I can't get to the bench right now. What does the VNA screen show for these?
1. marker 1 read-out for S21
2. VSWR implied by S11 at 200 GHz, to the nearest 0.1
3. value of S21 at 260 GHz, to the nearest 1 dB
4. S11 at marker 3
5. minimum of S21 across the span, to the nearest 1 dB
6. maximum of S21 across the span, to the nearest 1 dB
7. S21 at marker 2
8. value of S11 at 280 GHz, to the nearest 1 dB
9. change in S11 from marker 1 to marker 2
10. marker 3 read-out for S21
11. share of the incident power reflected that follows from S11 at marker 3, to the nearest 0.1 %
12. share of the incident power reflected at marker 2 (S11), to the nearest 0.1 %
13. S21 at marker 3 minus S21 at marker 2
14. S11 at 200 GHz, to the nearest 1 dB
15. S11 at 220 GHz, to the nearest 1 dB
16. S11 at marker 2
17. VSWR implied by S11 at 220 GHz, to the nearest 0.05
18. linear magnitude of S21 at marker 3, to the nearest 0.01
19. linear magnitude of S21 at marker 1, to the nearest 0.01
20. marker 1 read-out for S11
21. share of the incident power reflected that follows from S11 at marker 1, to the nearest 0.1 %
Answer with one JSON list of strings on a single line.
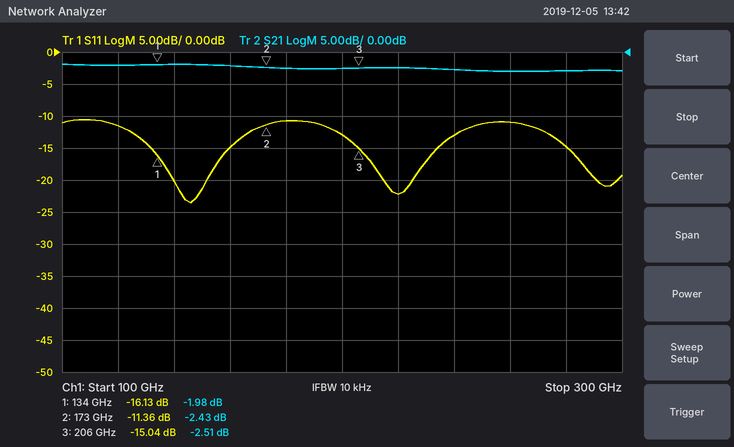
["-1.98 dB", "1.6", "-3 dB", "-15.04 dB", "-3 dB", "-2 dB", "-2.43 dB", "-15 dB", "4.77 dB", "-2.51 dB", "3.1 %", "7.3 %", "-0.08 dB", "-13 dB", "-22 dB", "-11.36 dB", "1.15", "0.75", "0.80", "-16.13 dB", "2.4 %"]
